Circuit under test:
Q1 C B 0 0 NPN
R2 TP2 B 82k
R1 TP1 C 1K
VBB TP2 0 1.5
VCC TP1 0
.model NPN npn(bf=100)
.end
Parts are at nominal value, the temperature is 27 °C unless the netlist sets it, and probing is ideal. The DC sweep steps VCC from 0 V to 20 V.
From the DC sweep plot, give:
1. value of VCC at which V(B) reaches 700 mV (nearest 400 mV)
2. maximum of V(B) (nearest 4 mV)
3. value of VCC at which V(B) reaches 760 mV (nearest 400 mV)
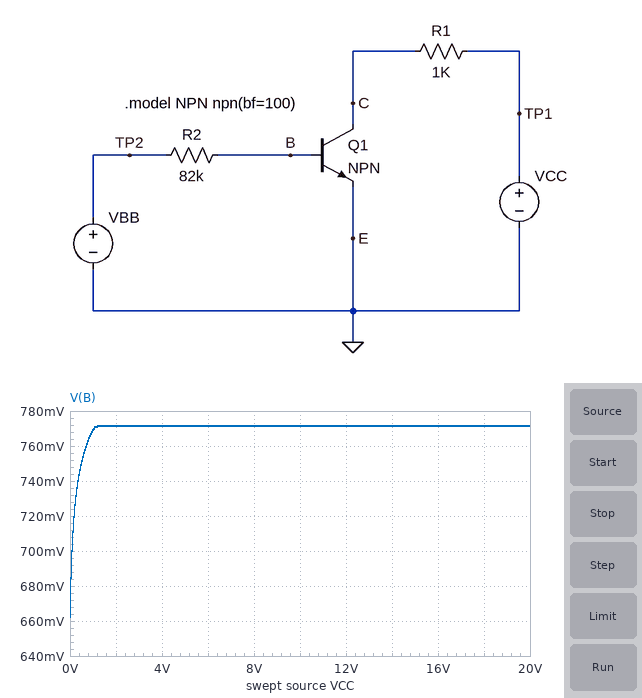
0 V
772 mV
800 mV
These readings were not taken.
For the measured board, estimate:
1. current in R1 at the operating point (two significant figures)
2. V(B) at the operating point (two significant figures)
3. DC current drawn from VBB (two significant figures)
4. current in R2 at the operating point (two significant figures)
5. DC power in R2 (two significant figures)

7.0 µA
660 mV
10 µA
10 µA
8.6 µW
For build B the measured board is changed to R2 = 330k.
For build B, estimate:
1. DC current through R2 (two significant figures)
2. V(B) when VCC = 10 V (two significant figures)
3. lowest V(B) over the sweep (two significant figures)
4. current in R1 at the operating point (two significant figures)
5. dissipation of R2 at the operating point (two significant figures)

2.7 µA
740 mV
620 mV
2.4 µA
2.3 µW
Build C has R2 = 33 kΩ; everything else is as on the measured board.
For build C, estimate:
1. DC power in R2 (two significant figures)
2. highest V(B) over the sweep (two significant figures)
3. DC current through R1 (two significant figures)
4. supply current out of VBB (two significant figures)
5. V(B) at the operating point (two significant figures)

20 µW
790 mV
11 µA
25 µA
690 mV
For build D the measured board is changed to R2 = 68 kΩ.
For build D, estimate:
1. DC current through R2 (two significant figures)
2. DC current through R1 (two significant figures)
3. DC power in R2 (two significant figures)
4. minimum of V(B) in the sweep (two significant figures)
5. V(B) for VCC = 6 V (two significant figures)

12 µA
7.8 µA
10 µW
670 mV
780 mV
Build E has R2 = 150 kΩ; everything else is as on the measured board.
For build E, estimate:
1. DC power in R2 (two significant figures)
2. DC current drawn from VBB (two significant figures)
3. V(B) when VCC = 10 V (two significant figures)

4.9 µW
5.7 µA
760 mV
